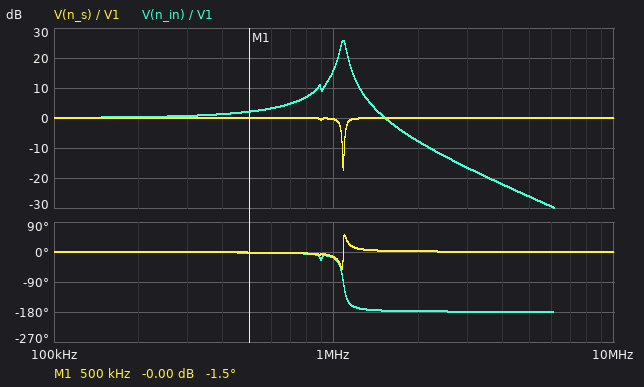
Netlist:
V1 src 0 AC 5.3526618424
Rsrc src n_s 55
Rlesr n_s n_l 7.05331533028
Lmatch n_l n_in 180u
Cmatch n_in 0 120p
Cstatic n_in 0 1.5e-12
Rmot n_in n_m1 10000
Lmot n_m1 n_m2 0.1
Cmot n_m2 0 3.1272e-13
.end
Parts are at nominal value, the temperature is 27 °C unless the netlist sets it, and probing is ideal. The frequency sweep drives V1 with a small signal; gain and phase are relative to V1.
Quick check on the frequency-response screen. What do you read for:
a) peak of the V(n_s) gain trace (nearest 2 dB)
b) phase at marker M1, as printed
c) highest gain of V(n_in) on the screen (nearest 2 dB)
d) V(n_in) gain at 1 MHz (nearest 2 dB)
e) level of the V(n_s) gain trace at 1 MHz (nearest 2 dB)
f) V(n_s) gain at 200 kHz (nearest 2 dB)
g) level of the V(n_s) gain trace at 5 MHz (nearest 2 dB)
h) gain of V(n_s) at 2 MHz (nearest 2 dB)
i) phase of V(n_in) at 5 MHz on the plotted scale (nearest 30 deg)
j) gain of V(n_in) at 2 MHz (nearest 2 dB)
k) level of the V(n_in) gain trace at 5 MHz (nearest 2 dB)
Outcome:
0 dB
-1.5 deg
26 dB
16 dB
0 dB
0 dB
0 dB
0 dB
-180 deg
-8 dB
-26 dB
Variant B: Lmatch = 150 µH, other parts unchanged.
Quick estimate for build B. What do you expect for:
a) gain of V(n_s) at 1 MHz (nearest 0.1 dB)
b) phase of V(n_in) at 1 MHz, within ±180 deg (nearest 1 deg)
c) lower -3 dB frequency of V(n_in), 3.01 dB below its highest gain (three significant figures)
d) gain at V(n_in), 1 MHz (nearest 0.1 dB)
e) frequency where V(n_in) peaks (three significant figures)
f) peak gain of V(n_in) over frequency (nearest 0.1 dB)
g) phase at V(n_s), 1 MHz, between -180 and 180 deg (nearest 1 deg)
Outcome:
-0.1 dB
-9 deg
1.15 MHz
10.7 dB
1.18 MHz
25.1 dB
-8 deg
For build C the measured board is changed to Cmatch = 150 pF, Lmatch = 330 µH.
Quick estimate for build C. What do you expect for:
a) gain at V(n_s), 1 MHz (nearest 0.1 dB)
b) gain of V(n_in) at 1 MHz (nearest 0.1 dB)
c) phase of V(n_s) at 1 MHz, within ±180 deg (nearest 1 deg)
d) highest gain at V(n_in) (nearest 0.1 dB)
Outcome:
0 dB
0.4 dB
3 deg
27.5 dB
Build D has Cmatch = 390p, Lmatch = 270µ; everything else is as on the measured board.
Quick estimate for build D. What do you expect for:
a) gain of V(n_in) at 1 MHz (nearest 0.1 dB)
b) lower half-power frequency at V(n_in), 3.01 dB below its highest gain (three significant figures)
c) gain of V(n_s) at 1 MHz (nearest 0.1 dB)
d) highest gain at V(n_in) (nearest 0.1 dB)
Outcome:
-10.0 dB
470 kHz
0 dB
22.5 dB
